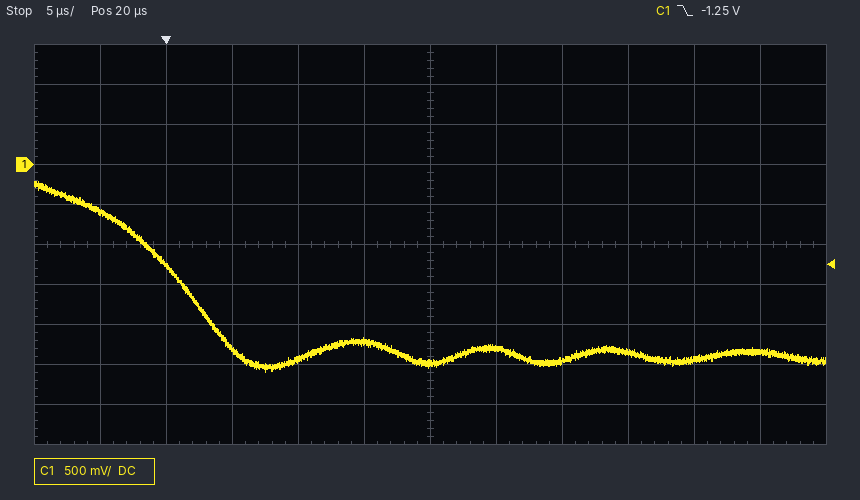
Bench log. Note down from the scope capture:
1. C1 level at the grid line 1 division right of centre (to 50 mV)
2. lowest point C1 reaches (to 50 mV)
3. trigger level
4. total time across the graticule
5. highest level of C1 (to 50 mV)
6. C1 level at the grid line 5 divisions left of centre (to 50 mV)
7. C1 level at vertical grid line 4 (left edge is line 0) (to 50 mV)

-2.30 V
-2.60 V
-1.25 V
60 µs
-200 mV
-600 mV
-2.45 V
